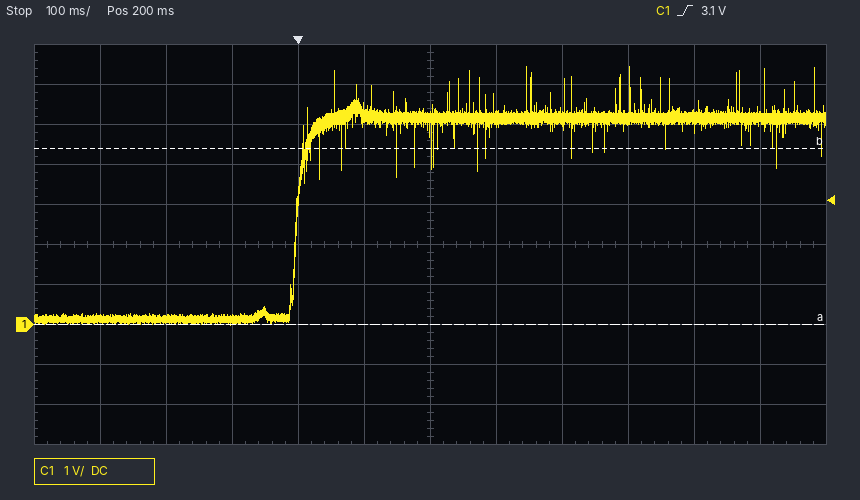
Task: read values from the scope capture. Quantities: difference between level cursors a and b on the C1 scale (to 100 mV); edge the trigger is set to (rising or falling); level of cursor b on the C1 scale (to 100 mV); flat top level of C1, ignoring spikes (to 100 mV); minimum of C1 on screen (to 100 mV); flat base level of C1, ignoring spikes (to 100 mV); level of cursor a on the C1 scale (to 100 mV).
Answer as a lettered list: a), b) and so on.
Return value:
a) 4.4 V
b) rising
c) 4.4 V
d) 5.2 V
e) 0.0 V
f) 100 mV
g) 0.0 V
